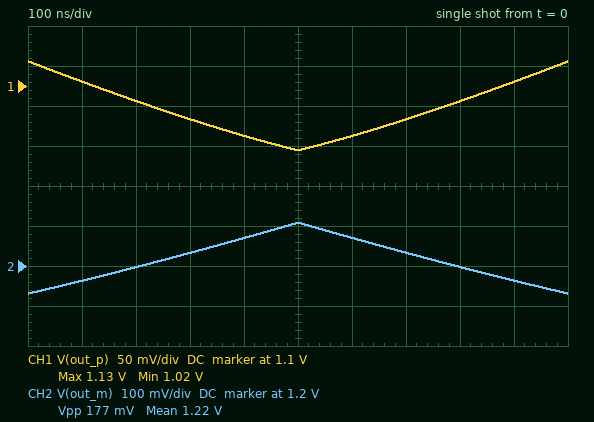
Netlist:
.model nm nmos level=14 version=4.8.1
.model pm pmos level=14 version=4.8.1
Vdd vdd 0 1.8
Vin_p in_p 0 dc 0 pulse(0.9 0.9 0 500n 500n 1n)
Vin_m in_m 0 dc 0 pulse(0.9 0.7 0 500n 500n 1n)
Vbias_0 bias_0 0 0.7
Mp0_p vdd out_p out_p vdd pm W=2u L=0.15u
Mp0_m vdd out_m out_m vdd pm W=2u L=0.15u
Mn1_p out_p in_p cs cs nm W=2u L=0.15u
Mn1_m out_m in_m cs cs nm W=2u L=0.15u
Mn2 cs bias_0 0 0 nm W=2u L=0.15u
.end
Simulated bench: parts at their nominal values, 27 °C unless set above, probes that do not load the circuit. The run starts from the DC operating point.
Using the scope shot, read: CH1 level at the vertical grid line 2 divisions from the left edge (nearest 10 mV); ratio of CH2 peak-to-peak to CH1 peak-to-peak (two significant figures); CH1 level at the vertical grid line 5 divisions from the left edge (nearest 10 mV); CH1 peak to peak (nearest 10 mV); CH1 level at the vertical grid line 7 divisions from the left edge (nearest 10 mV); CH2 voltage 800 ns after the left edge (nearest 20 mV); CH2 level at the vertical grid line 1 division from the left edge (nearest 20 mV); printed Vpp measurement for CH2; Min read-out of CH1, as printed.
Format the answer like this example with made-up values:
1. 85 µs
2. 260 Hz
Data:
1. 1.08 V
2. 1.6
3. 1.02 V
4. 110 mV
5. 1.06 V
6. 1.20 V
7. 1.16 V
8. 177 mV
9. 1.02 V
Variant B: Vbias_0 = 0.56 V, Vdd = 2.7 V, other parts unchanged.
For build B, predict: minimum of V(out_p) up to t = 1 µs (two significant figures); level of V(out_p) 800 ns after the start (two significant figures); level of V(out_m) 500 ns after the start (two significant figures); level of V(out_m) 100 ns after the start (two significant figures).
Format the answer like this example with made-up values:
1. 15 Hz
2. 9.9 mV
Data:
1. 2.0 V
2. 2.1 V
3. 2.3 V
4. 2.2 V
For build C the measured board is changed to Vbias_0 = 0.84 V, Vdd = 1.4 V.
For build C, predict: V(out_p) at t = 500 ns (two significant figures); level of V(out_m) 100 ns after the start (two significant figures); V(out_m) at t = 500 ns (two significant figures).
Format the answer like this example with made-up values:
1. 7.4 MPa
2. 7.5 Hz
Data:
1. 580 mV
2. 690 mV
3. 820 mV
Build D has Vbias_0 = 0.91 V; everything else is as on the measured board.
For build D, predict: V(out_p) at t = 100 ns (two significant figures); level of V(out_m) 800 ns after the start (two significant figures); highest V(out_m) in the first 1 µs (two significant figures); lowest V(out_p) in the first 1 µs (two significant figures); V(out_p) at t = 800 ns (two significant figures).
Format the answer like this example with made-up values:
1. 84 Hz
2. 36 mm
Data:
1. 1.0 V
2. 1.1 V
3. 1.2 V
4. 930 mV
5. 980 mV
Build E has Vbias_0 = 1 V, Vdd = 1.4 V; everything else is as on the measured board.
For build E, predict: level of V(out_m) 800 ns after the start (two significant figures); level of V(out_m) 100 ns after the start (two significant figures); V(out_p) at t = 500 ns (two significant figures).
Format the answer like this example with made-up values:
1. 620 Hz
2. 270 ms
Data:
1. 660 mV
2. 630 mV
3. 540 mV
